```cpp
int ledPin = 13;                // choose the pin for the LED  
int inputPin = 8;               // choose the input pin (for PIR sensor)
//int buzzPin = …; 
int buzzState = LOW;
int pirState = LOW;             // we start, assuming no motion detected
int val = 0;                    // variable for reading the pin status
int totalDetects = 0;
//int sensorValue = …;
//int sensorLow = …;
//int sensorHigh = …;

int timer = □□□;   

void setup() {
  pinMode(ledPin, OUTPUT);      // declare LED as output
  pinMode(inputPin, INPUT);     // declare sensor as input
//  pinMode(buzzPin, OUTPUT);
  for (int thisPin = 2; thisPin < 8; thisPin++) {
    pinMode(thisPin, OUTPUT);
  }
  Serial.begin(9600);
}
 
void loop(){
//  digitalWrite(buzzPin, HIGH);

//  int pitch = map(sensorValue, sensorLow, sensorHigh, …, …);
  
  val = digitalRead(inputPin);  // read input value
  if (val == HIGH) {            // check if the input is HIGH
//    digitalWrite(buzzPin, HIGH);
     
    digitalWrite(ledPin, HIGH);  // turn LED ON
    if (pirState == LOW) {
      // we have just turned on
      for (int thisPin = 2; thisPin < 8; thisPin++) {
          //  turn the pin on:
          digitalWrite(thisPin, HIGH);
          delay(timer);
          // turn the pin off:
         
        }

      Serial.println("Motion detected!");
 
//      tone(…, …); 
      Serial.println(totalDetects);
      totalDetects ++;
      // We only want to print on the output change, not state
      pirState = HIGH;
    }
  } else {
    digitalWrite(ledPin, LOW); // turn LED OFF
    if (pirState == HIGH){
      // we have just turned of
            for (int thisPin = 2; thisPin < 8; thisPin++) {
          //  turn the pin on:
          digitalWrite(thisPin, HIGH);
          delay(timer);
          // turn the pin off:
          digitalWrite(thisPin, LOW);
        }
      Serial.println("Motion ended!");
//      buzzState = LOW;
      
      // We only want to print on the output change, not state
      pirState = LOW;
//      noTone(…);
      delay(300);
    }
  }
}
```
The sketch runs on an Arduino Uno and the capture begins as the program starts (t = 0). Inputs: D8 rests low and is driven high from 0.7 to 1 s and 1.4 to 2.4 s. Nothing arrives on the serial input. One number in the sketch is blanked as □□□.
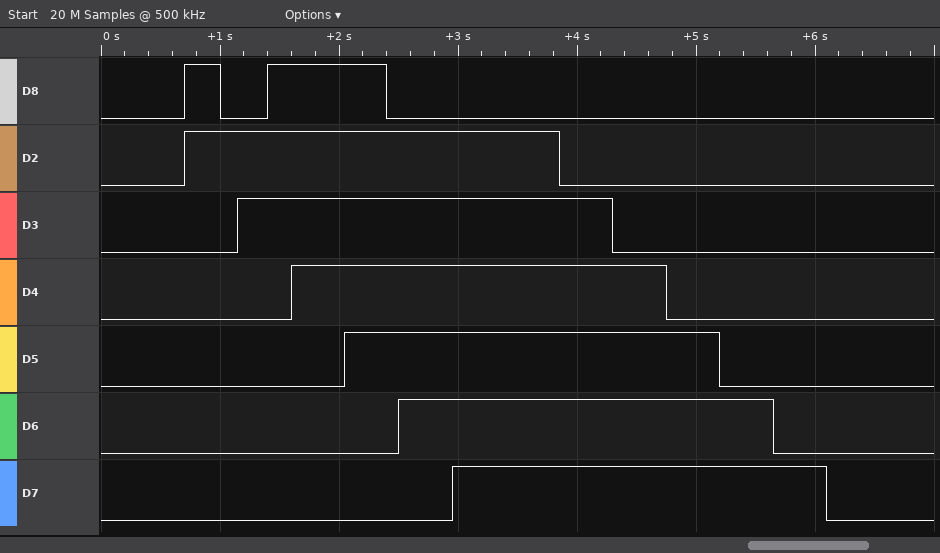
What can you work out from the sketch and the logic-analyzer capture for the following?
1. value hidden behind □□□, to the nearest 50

450
